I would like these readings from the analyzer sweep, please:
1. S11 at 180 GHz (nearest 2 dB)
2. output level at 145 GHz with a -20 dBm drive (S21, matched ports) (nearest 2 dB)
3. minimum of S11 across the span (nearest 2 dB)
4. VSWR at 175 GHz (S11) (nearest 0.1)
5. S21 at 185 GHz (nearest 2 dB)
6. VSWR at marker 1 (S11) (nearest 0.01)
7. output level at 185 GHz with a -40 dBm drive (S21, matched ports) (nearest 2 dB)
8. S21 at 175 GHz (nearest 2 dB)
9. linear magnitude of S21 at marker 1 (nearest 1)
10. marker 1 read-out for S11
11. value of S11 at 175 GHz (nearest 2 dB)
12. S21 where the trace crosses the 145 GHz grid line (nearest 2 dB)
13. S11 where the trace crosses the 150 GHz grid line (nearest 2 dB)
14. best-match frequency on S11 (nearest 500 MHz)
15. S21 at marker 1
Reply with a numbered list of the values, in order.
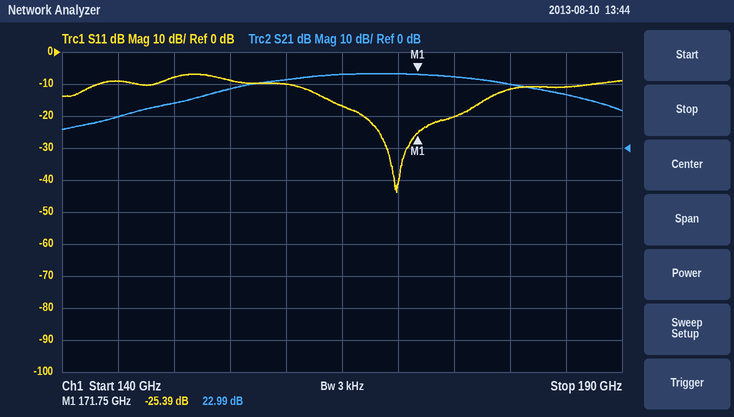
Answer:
1. -12 dB
2. -10 dBm
3. -44 dB
4. 1.2
5. 16 dB
6. 1.11
7. -24 dBm
8. 22 dB
9. 14
10. -25.39 dB
11. -20 dB
12. 10 dB
13. -8 dB
14. 170.0 GHz
15. 22.99 dB
